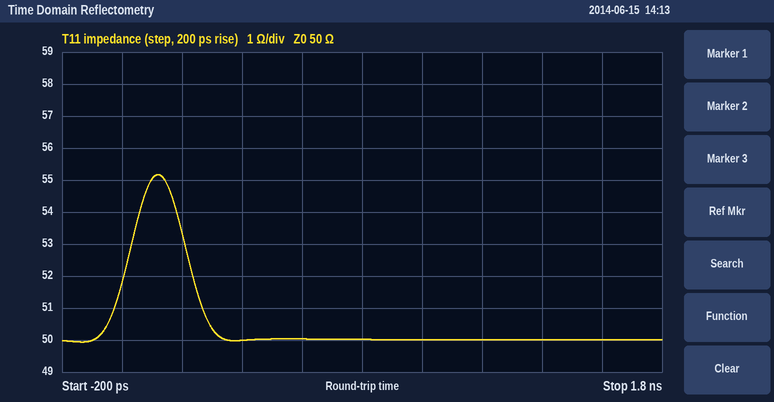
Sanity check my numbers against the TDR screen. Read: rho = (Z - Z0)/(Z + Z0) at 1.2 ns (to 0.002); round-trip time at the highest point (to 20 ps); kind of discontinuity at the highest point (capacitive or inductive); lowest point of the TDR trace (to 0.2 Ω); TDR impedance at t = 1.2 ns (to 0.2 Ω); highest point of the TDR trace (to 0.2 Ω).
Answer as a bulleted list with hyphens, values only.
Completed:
- 0.000
- 120 ps
- inductive
- 50.0 Ω
- 50.0 Ω
- 55.2 Ω
